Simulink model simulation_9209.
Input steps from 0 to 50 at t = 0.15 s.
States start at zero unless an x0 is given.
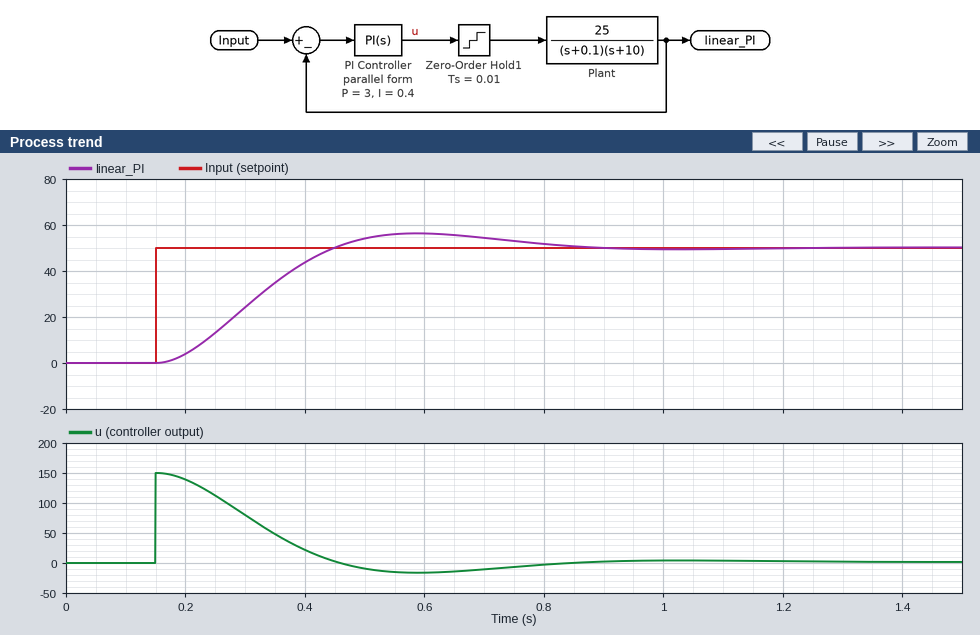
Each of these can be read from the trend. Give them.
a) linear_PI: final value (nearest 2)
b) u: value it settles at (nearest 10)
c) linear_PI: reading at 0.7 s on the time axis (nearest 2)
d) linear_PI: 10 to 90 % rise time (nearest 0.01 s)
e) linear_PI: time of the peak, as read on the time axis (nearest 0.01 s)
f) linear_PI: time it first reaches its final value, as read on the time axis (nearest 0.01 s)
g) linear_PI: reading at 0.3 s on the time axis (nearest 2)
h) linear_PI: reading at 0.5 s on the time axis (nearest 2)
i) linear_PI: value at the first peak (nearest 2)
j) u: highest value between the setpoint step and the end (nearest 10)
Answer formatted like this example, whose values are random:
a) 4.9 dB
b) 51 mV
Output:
a) 50
b) 0
c) 54
d) 0.20 s
e) 0.59 s
f) 0.45 s
g) 24
h) 54
i) 56
j) 150
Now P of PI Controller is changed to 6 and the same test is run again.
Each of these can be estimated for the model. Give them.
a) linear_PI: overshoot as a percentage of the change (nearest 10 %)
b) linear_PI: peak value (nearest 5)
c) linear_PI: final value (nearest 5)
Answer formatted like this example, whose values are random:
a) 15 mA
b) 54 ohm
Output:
a) 30 %
b) 65
c) 50
